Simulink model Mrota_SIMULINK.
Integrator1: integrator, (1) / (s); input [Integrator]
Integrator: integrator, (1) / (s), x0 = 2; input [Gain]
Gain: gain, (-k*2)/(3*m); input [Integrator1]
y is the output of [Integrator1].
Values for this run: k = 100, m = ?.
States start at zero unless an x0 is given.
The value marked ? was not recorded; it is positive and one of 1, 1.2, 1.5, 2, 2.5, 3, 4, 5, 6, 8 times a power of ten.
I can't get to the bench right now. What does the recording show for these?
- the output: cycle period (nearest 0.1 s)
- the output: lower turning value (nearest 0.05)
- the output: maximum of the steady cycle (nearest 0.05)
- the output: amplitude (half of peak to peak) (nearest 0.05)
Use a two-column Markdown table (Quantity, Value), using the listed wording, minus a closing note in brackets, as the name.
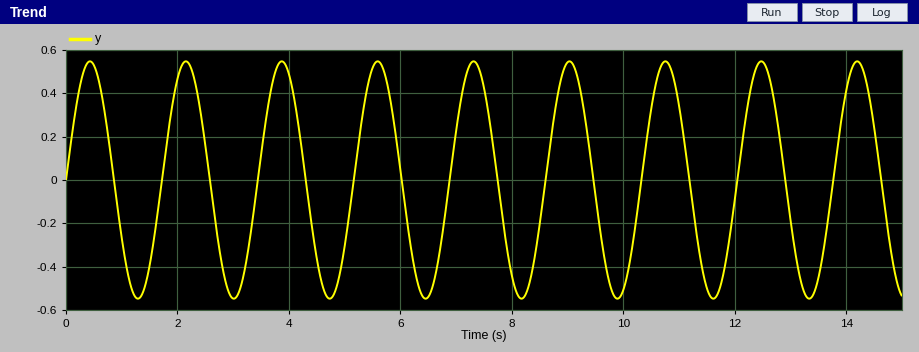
| Quantity | Value |
|---|---|
| the output: cycle period | 1.7 s |
| the output: lower turning value | -0.55 |
| the output: maximum of the steady cycle | 0.55 |
| the output: amplitude (half of peak to peak) | 0.55 |
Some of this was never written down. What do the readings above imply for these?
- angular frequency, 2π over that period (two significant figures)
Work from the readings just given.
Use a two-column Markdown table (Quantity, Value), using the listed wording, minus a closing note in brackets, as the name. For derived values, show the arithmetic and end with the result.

| Quantity | Value |
|---|---|
| angular frequency, 2π over that period | 2π / 1.7 = 3.7 rad/s |
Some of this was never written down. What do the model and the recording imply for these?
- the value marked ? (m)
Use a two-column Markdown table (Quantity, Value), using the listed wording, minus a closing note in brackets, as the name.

| Quantity | Value |
|---|---|
| the value marked ? | 5 |
